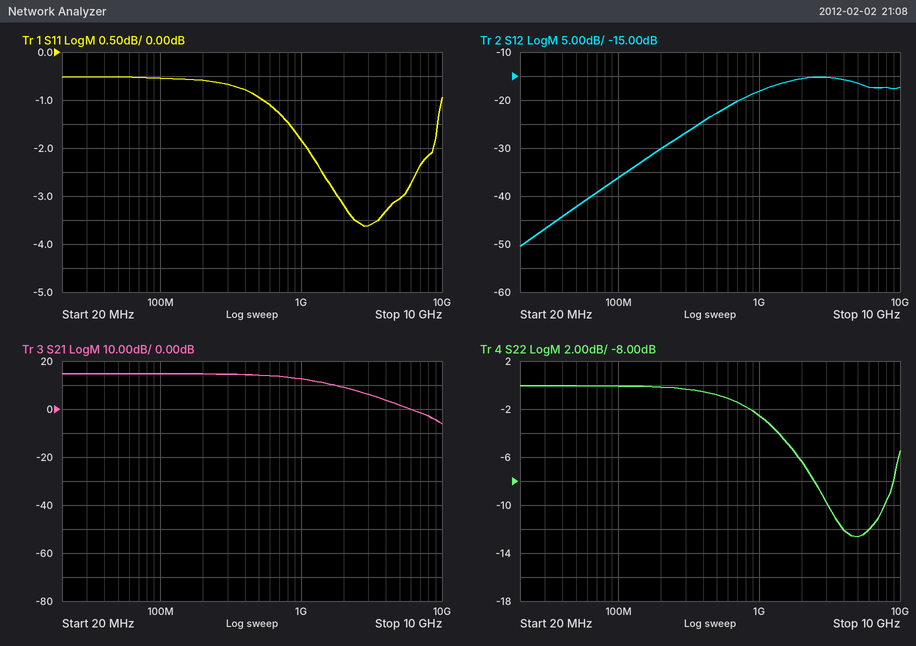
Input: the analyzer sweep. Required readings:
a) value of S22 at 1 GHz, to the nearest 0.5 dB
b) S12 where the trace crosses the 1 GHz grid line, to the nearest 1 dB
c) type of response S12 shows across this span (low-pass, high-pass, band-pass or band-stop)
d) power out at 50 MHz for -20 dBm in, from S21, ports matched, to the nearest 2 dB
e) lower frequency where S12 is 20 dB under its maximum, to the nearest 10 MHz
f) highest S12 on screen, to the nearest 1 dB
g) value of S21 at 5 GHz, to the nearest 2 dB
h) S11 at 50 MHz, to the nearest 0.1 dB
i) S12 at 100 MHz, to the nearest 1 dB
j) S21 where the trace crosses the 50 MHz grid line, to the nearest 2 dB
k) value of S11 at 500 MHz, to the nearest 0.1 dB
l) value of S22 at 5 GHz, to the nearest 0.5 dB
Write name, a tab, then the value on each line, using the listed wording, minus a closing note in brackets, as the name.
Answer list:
value of S22 at 1 GHz, to the nearest 0.5 dB	-2.5 dB
S12 where the trace crosses the 1 GHz grid line, to the nearest 1 dB	-18 dB
type of response S12 shows across this span	high-pass
power out at 50 MHz for -20 dBm in, from S21, ports matched, to the nearest 2 dB	-6 dBm
lower frequency where S12 is 20 dB under its maximum, to the nearest 10 MHz	110 MHz
highest S12 on screen, to the nearest 1 dB	-15 dB
value of S21 at 5 GHz, to the nearest 2 dB	2 dB
S11 at 50 MHz, to the nearest 0.1 dB	-0.5 dB
S12 at 100 MHz, to the nearest 1 dB	-36 dB
S21 where the trace crosses the 50 MHz grid line, to the nearest 2 dB	14 dB
value of S11 at 500 MHz, to the nearest 0.1 dB	-0.9 dB
value of S22 at 5 GHz, to the nearest 0.5 dB	-12.5 dB
